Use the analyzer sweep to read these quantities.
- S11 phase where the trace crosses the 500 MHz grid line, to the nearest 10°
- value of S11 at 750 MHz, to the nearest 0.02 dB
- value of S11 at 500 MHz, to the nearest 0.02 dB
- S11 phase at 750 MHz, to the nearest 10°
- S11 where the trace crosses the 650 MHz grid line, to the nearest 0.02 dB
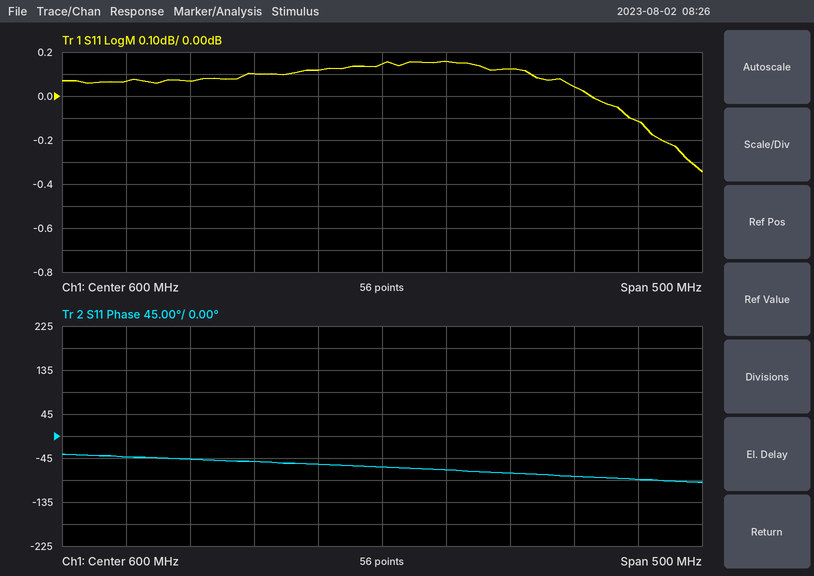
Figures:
-50°
0.04 dB
0.10 dB
-80°
0.16 dB
